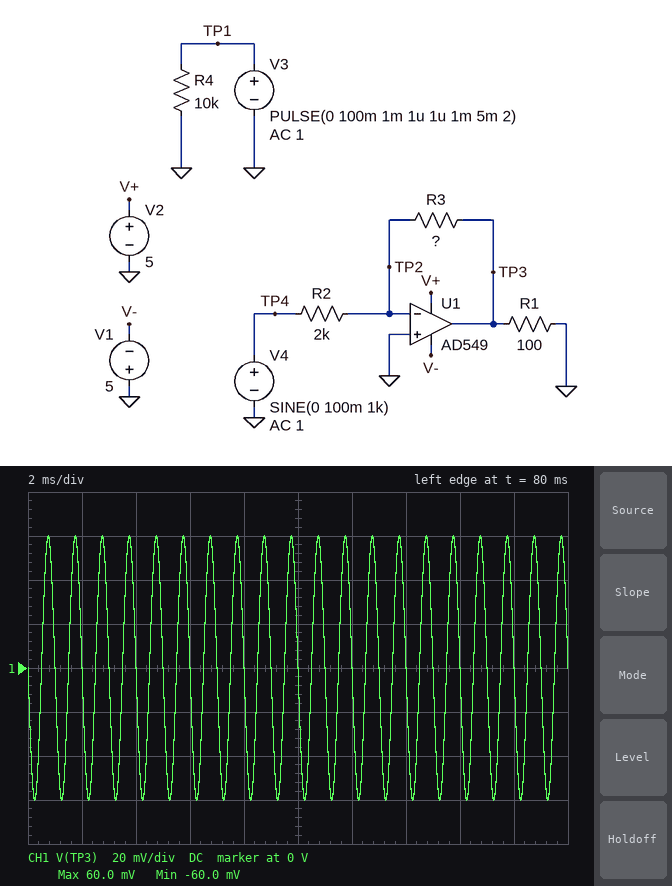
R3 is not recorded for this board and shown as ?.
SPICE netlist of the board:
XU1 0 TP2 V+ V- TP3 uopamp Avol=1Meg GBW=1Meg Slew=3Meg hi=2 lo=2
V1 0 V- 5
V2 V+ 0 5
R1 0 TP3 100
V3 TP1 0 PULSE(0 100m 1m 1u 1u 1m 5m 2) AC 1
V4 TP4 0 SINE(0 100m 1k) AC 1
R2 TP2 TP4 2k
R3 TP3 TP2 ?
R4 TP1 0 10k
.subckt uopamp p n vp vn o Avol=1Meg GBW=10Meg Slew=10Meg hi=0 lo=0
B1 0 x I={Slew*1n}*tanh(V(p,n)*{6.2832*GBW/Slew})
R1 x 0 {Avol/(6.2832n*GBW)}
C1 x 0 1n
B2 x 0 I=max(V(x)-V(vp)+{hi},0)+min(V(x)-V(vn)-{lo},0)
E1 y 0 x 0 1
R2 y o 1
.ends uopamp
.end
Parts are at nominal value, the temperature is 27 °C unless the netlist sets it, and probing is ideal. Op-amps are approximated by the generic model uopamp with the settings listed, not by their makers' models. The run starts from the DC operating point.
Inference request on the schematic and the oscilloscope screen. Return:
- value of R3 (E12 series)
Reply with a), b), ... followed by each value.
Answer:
a) 1.2 kΩ
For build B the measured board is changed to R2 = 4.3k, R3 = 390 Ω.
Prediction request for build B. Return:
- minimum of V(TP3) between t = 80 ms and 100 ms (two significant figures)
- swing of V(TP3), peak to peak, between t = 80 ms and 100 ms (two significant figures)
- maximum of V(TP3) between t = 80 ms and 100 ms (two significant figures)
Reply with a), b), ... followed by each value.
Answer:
a) -9.1 mV
b) 18 mV
c) 9.1 mV
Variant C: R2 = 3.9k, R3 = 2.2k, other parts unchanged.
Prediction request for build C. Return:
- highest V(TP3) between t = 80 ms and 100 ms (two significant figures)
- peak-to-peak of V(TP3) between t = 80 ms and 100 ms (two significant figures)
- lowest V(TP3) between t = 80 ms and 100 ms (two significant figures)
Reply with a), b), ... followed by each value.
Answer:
a) 56 mV
b) 110 mV
c) -56 mV
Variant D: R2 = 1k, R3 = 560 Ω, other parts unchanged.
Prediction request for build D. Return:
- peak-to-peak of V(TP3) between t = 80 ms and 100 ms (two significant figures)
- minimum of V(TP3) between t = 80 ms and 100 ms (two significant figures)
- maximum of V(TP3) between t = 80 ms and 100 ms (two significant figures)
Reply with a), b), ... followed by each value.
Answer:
a) 110 mV
b) -56 mV
c) 56 mV
